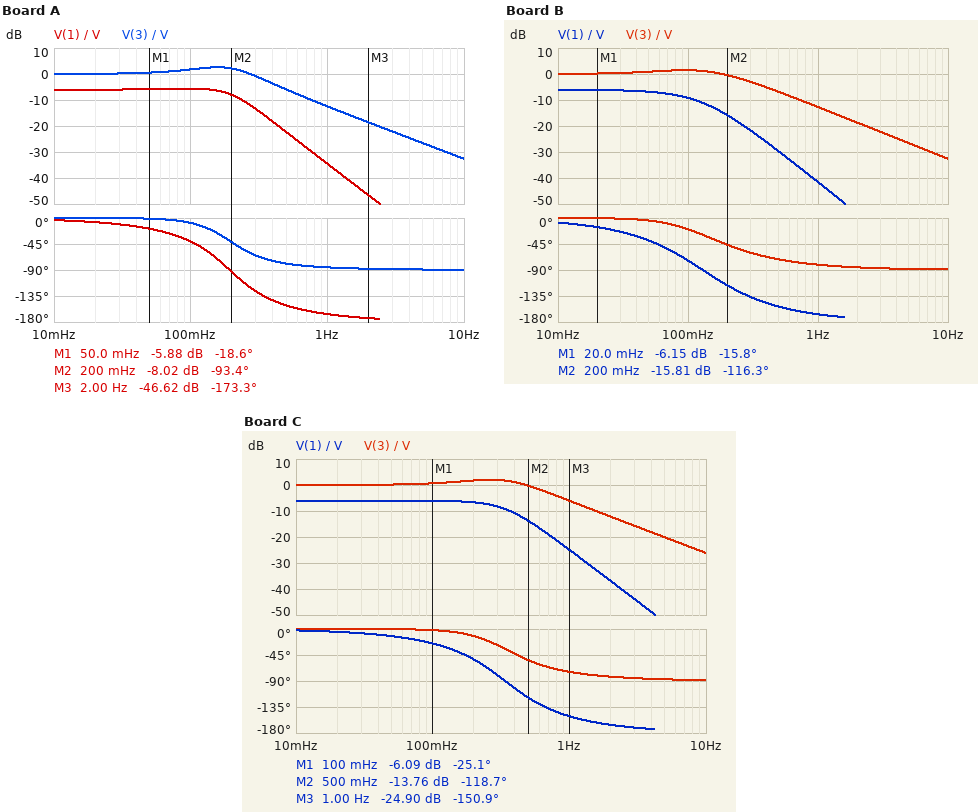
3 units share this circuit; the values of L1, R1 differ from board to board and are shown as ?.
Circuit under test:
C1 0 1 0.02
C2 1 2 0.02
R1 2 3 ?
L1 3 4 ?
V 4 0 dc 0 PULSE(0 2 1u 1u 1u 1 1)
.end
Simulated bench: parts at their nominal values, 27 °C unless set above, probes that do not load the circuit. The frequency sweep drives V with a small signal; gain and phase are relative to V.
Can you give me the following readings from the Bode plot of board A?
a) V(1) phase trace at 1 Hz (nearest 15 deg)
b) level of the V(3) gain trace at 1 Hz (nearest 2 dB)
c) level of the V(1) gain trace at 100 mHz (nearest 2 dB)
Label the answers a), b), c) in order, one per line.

a) -165 deg
b) -12 dB
c) -6 dB
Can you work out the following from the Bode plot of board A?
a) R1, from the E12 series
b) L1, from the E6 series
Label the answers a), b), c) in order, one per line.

a) 100 Ω
b) 68 H
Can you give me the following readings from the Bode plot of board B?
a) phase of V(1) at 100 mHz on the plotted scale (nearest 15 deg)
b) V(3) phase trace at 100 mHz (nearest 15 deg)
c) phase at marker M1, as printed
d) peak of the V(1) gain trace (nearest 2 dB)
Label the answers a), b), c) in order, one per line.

a) -75 deg
b) -15 deg
c) -15.8 deg
d) -6 dB
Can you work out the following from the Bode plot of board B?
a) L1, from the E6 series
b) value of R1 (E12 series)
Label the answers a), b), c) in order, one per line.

a) 150 H
b) 220 Ω
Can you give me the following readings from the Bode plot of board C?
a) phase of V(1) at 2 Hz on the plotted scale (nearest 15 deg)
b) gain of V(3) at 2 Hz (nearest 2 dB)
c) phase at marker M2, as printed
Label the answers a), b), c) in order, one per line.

a) -165 deg
b) -12 dB
c) -118.7 deg
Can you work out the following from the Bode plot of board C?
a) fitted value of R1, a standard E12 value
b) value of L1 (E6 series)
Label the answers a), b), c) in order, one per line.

a) 68 Ω
b) 22 H
